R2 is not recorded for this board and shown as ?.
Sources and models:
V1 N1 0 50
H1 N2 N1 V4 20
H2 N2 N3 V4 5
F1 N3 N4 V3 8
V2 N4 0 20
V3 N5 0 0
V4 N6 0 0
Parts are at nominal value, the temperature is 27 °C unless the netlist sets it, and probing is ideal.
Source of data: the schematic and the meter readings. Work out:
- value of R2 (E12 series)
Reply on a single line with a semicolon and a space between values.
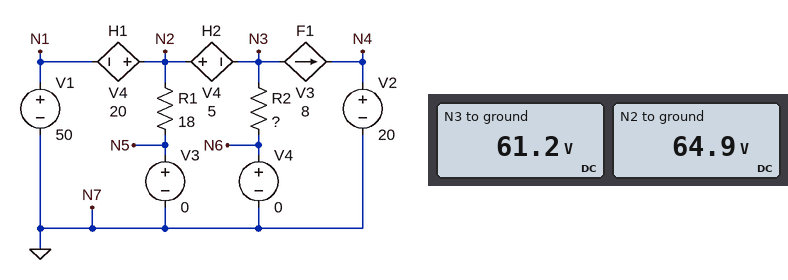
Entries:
82 Ω
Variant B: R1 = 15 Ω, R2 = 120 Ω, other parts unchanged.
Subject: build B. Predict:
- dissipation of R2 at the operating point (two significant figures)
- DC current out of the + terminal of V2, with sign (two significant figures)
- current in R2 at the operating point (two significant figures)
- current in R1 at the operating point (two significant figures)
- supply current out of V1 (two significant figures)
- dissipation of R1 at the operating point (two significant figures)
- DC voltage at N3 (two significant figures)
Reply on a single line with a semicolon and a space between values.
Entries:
27 W; -32 A; 480 mA; 4.0 A; 36 A; 240 W; 57 V
